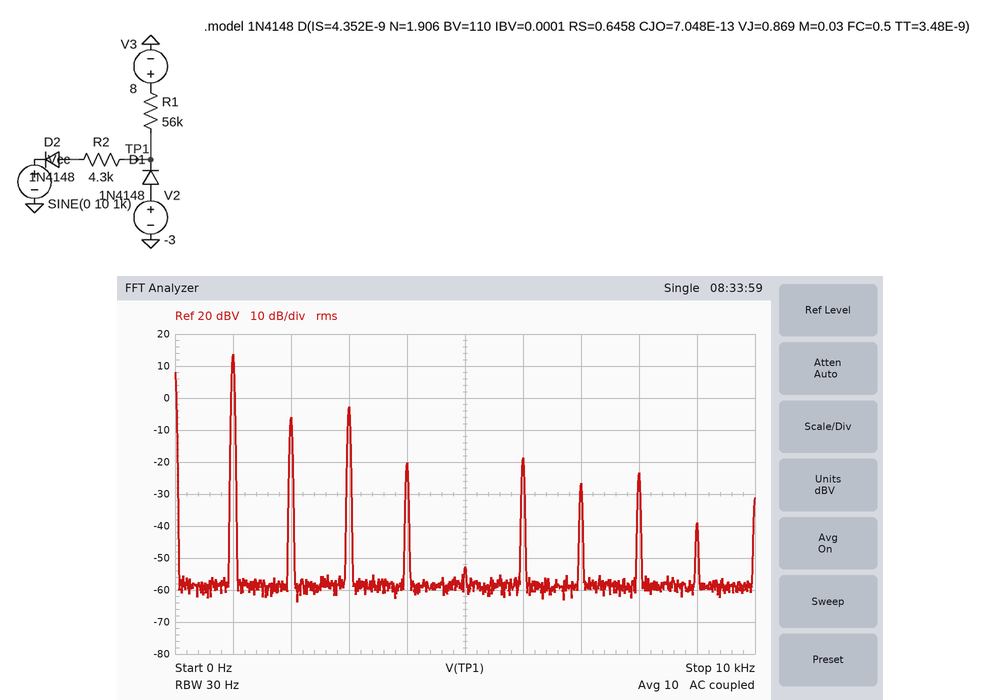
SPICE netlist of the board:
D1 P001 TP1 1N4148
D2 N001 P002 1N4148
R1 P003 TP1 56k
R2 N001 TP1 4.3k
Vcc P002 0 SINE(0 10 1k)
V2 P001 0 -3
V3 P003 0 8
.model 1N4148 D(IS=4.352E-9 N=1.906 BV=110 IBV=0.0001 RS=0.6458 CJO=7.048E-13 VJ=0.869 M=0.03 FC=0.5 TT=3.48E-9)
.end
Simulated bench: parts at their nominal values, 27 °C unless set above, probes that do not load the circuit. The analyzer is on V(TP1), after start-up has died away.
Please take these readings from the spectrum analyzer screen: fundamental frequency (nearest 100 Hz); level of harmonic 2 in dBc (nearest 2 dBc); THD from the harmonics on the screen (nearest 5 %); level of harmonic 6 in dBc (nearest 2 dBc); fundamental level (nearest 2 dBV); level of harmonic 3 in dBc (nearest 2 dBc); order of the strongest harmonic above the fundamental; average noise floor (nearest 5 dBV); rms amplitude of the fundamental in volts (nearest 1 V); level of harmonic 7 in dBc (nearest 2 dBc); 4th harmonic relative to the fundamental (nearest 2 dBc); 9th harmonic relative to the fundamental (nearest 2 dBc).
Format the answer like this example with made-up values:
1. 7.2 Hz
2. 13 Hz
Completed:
1. 1.0 kHz
2. -20 dBc
3. 20 %
4. -32 dBc
5. 14 dBV
6. -16 dBc
7. 3
8. -60 dBV
9. 5 V
10. -40 dBc
11. -34 dBc
12. -52 dBc
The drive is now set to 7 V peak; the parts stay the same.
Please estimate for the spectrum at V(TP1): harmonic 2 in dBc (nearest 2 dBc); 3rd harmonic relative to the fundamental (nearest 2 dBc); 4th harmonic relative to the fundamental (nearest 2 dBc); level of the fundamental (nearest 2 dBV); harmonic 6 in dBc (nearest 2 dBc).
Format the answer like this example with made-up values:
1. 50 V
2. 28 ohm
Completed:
1. -22 dBc
2. -24 dBc
3. -30 dBc
4. 12 dBV
5. -50 dBc
